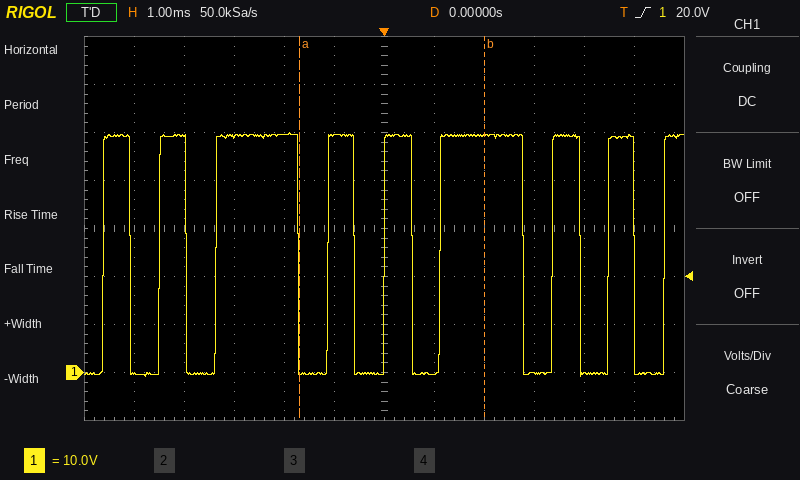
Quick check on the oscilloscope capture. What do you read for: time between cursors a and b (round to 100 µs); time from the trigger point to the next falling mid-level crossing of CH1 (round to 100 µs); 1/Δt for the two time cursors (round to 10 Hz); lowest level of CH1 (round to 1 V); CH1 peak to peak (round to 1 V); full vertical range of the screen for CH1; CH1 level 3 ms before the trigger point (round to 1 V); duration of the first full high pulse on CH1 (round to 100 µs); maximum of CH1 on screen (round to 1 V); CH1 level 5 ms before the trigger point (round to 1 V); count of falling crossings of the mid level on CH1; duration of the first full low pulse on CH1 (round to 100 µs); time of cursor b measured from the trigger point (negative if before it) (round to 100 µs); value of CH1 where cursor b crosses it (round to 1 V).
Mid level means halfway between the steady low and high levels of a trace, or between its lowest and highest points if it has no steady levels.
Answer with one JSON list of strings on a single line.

["3.7 ms", "600 µs", "270 Hz", "-1 V", "51 V", "80 V", "49 V", "500 µs", "50 V", "0 V", "8", "600 µs", "+2.0 ms", "49 V"]
